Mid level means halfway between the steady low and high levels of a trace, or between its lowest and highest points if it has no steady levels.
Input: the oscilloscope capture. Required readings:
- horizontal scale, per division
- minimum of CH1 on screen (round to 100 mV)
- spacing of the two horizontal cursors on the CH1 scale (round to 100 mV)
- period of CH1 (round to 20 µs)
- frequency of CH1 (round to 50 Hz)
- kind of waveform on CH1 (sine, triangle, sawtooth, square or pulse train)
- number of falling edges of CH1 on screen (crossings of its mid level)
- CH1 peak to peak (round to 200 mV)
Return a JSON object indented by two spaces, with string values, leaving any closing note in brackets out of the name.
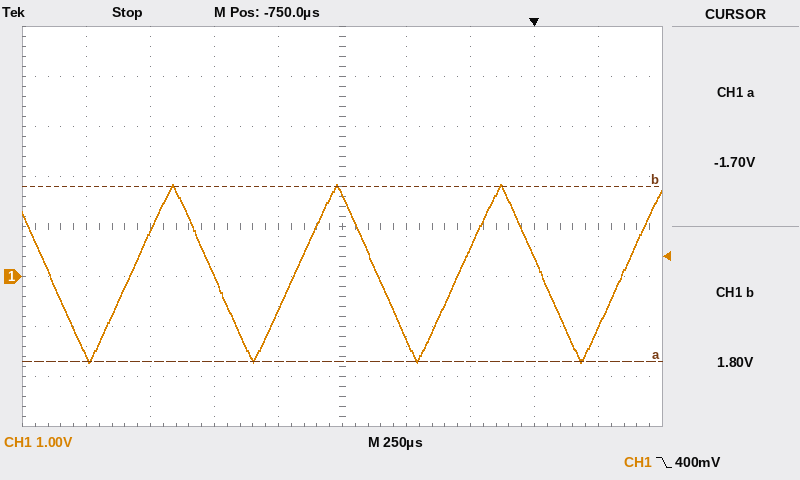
{
  "horizontal scale, per division": "250 µs",
  "minimum of CH1 on screen": "-1.7 V",
  "spacing of the two horizontal cursors on the CH1 scale": "3.5 V",
  "period of CH1": "640 µs",
  "frequency of CH1": "1.55 kHz",
  "kind of waveform on CH1": "triangle",
  "number of falling edges of CH1 on screen": "4",
  "CH1 peak to peak": "3.6 V"
}
